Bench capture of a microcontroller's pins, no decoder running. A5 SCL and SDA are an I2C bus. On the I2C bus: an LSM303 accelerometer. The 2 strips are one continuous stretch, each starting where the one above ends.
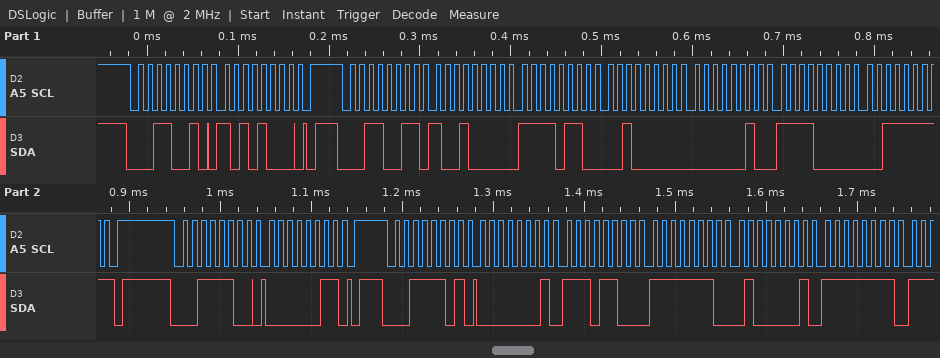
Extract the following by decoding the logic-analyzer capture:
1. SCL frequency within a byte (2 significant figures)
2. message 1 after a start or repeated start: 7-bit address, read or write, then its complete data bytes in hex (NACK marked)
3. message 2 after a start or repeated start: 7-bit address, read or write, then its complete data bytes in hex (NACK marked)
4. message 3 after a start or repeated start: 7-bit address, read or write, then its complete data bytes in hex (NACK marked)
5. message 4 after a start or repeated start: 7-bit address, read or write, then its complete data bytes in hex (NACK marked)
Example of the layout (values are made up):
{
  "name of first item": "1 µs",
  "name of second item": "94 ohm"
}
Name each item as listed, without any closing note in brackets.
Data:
{
  "SCL frequency within a byte": "100 kHz",
  "message 1 after a start or repeated start: 7-bit address, read or write, then its complete data bytes in hex": "0x19 write: A8",
  "message 2 after a start or repeated start: 7-bit address, read or write, then its complete data bytes in hex": "0x19 read: 90 F6 20 02 F0 3F NACK",
  "message 3 after a start or repeated start: 7-bit address, read or write, then its complete data bytes in hex": "0x1E write: 03",
  "message 4 after a start or repeated start: 7-bit address, read or write, then its complete data bytes in hex": "0x1E read: 01 EC FE 41 FF"
}
